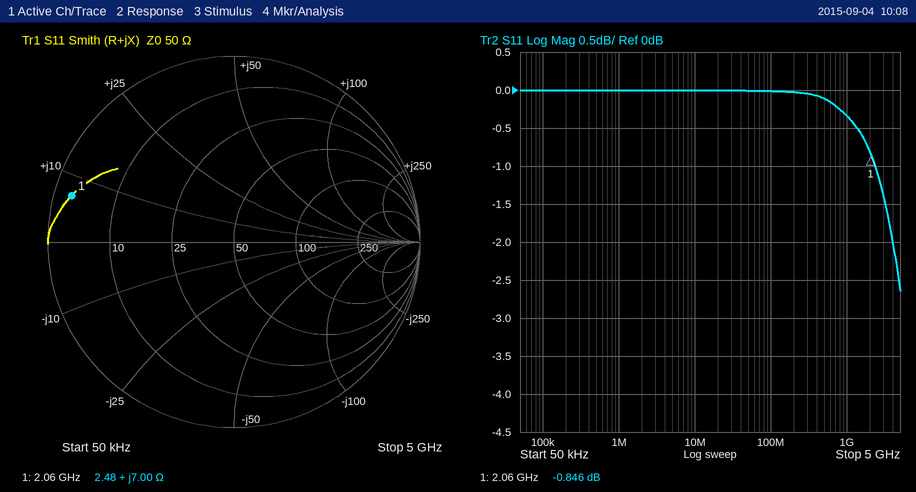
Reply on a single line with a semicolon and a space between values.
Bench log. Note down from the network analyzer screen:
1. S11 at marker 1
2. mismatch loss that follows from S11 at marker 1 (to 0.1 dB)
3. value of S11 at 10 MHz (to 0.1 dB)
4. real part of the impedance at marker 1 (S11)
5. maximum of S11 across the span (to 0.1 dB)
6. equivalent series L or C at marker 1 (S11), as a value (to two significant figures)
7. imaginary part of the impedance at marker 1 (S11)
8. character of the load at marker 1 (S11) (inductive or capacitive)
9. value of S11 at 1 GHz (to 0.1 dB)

-0.846 dB; 7.5 dB; 0.0 dB; 2.48 Ω; 0.0 dB; 540 pH; +7.00 Ω; inductive; -0.3 dB
